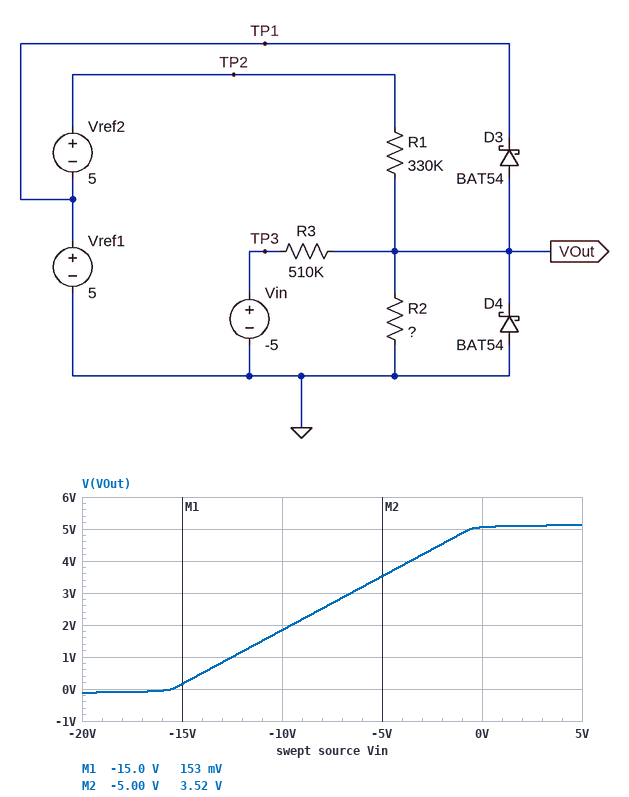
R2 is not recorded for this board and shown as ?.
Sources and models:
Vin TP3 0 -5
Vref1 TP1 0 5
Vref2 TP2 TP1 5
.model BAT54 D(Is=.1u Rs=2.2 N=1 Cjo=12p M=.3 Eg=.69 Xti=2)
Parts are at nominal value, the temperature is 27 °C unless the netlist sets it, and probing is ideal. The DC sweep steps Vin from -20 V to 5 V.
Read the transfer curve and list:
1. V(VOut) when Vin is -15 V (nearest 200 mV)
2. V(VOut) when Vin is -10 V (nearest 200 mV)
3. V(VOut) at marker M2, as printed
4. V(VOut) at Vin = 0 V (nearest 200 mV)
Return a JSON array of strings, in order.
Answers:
["200 mV", "1.8 V", "3.52 V", "5.0 V"]
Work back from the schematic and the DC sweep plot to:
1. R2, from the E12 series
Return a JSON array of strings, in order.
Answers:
["1.2 MΩ"]
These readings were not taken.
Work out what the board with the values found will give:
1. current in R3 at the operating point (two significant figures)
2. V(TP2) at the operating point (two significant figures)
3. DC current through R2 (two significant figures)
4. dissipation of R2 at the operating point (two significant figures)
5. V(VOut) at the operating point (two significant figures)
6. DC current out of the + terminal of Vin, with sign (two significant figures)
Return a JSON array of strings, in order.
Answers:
["17 µA", "10 V", "2.9 µA", "10 µW", "3.5 V", "-17 µA"]
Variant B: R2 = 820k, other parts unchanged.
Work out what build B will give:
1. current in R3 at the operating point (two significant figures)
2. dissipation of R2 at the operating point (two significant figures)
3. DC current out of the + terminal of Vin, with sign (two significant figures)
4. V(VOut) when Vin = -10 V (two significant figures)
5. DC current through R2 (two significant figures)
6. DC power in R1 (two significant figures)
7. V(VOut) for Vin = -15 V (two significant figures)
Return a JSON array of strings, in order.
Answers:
["16 µA", "13 µW", "-16 µA", "1.7 V", "4.0 µA", "140 µW", "140 mV"]
